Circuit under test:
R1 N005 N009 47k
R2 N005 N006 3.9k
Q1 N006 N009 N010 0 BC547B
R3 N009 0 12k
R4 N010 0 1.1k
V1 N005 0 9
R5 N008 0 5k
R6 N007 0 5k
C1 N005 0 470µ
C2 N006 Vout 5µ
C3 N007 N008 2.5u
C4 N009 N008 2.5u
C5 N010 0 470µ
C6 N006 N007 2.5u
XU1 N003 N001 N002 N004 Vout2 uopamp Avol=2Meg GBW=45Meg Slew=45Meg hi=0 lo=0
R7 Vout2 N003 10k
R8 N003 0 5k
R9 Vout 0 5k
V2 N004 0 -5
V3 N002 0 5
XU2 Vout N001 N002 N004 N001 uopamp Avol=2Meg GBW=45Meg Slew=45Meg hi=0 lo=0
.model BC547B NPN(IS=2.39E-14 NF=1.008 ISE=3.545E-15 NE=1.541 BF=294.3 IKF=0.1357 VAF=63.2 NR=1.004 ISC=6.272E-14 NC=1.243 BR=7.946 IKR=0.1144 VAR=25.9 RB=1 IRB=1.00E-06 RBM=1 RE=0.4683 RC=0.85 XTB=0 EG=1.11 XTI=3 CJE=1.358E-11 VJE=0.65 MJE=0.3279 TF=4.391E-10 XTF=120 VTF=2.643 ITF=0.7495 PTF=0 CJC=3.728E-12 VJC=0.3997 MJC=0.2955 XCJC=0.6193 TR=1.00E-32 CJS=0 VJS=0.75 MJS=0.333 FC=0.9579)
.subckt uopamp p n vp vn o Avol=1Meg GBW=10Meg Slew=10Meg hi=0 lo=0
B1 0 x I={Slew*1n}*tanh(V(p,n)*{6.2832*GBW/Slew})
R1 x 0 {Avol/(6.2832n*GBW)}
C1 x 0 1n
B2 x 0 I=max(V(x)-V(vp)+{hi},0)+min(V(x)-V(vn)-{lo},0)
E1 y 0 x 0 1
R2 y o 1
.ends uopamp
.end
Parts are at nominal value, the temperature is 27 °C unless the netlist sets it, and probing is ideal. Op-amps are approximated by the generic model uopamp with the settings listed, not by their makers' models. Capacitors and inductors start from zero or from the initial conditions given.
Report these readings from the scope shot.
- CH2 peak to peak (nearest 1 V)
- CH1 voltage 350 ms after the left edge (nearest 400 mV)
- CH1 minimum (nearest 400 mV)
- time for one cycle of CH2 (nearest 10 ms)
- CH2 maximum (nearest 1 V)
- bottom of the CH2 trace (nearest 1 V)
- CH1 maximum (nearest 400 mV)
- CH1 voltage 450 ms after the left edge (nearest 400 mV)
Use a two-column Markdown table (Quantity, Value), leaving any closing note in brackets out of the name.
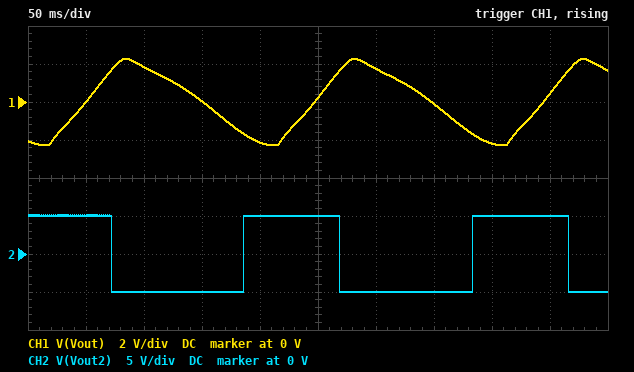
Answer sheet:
| Quantity | Value |
|---|---|
| CH2 peak to peak | 10 V |
| CH1 voltage 350 ms after the left edge | 0 V |
| CH1 minimum | -2.4 V |
| time for one cycle of CH2 | 200 ms |
| CH2 maximum | 5 V |
| bottom of the CH2 trace | -5 V |
| CH1 maximum | 2.4 V |
| CH1 voltage 450 ms after the left edge | 400 mV |
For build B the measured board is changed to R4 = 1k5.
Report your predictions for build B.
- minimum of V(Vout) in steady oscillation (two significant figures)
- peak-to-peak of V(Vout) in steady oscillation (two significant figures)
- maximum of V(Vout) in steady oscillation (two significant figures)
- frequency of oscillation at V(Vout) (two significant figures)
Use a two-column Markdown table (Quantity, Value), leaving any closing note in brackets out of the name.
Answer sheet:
| Quantity | Value |
|---|---|
| minimum of V(Vout) in steady oscillation | -1.4 V |
| peak-to-peak of V(Vout) in steady oscillation | 3.2 V |
| maximum of V(Vout) in steady oscillation | 1.7 V |
| frequency of oscillation at V(Vout) | 4.7 Hz |
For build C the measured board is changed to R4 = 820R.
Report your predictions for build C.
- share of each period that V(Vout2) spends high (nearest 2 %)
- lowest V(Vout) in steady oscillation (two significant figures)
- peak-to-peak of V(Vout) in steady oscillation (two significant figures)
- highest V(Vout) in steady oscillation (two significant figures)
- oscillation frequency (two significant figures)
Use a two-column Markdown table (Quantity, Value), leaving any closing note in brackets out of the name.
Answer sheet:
| Quantity | Value |
|---|---|
| share of each period that V(Vout2) spends high | 58 % |
| lowest V(Vout) in steady oscillation | -2.6 V |
| peak-to-peak of V(Vout) in steady oscillation | 4.3 V |
| highest V(Vout) in steady oscillation | 1.7 V |
| oscillation frequency | 5.5 Hz |
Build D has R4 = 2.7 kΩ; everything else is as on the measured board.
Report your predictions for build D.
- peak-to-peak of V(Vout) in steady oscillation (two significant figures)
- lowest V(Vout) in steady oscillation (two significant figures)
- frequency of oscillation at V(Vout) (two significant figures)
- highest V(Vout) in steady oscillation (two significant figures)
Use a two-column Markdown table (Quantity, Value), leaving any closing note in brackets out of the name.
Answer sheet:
| Quantity | Value |
|---|---|
| peak-to-peak of V(Vout) in steady oscillation | 1.4 V |
| lowest V(Vout) in steady oscillation | -660 mV |
| frequency of oscillation at V(Vout) | 5.0 Hz |
| highest V(Vout) in steady oscillation | 770 mV |
